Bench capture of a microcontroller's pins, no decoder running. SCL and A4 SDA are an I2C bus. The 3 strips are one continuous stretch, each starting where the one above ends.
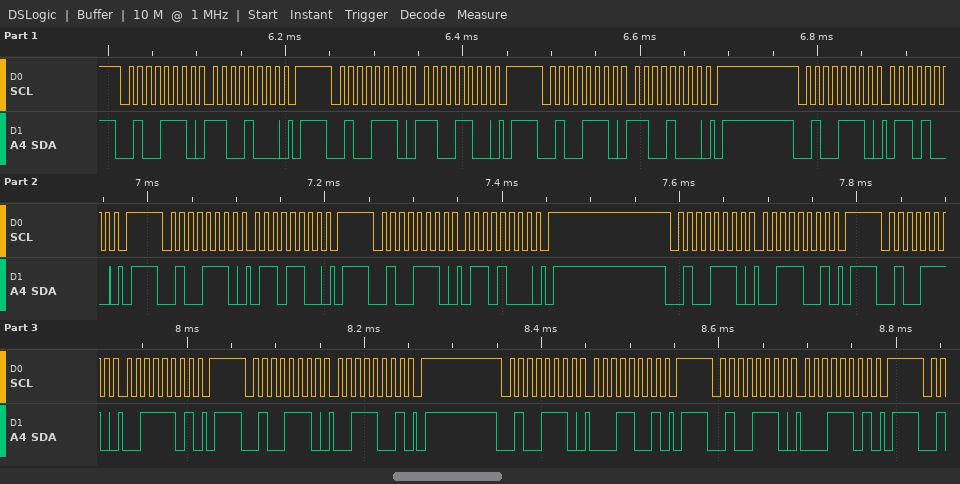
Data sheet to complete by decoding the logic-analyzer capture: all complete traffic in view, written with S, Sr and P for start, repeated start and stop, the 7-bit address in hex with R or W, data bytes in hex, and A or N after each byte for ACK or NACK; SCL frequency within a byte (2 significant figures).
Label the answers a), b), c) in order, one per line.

a) S 27W A C8 A P S 27W A CC A P S 27W A C8 A P S 27W A 68 A P S 27W A 6C A P S 27W A 68 A P S 27W A 39 A P S 27W A 3D A P S 27W A 39 A P S 27W A 19 A P S 27W A 1D A P
b) 100 kHz
